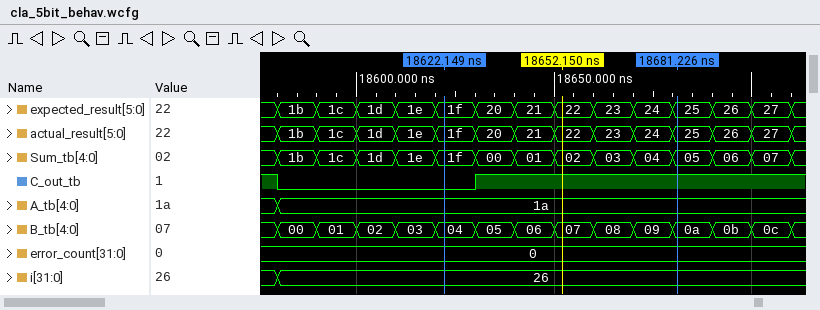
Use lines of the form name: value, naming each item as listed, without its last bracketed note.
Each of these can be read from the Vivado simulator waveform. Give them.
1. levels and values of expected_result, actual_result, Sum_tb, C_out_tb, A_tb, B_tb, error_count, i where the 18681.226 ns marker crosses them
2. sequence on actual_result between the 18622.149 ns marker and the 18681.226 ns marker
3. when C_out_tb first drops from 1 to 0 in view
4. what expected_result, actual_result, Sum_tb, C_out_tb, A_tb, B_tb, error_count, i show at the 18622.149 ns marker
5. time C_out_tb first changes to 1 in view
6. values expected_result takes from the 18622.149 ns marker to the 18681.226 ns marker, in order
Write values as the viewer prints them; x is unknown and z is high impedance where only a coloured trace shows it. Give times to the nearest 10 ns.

levels and values of expected_result, actual_result, Sum_tb, C_out_tb, A_tb, B_tb, error_count, i where the 18681.226 ns marker crosses them: expected_result=25, actual_result=25, Sum_tb=05, C_out_tb=1, A_tb=1a, B_tb=0a, error_count=0, i=26
sequence on actual_result between the 18622.149 ns marker and the 18681.226 ns marker: 1f, 20, 21, 22, 23, 24, 25
when C_out_tb first drops from 1 to 0 in view: 18580 ns
what expected_result, actual_result, Sum_tb, C_out_tb, A_tb, B_tb, error_count, i show at the 18622.149 ns marker: expected_result=1f, actual_result=1f, Sum_tb=1f, C_out_tb=0, A_tb=1a, B_tb=04, error_count=0, i=26
time C_out_tb first changes to 1 in view: 18630 ns
values expected_result takes from the 18622.149 ns marker to the 18681.226 ns marker, in order: 1f, 20, 21, 22, 23, 24, 25
